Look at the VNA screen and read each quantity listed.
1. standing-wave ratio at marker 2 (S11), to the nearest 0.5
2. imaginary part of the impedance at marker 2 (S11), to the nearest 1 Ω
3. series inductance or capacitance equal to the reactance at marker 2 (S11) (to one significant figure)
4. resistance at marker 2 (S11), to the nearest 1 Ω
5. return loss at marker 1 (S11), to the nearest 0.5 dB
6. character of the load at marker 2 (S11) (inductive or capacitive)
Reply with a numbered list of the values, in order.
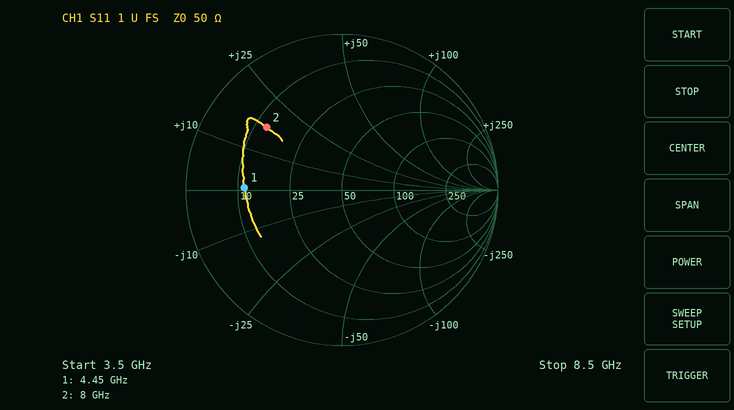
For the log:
1. 4.5
2. +17 Ω
3. 300 pH
4. 13 Ω
5. 4.0 dB
6. inductive
